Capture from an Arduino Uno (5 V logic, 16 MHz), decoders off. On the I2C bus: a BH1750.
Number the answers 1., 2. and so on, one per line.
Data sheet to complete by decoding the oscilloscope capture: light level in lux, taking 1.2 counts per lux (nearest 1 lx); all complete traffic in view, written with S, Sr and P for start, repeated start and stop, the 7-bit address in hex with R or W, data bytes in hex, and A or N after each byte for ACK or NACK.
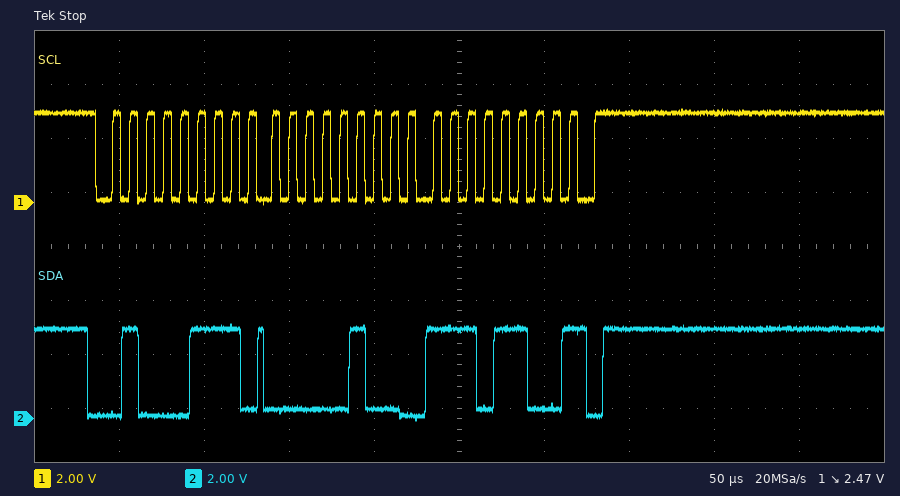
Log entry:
1. 1050 lx
2. S 23R A 04 A EC N P
